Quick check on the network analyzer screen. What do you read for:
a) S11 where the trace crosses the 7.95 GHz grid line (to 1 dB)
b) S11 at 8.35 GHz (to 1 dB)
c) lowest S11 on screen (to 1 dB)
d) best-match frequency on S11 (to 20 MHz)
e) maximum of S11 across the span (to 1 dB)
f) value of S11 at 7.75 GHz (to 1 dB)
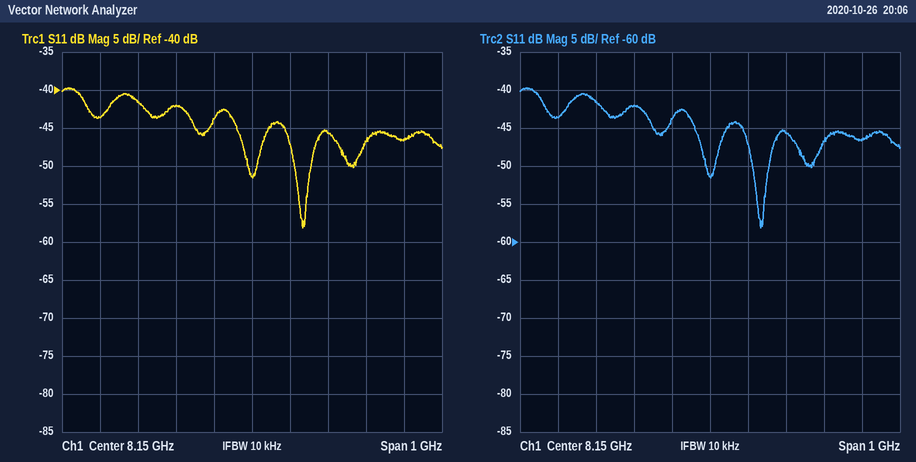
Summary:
-42 dB
-46 dB
-58 dB
8.28 GHz
-40 dB
-44 dB
